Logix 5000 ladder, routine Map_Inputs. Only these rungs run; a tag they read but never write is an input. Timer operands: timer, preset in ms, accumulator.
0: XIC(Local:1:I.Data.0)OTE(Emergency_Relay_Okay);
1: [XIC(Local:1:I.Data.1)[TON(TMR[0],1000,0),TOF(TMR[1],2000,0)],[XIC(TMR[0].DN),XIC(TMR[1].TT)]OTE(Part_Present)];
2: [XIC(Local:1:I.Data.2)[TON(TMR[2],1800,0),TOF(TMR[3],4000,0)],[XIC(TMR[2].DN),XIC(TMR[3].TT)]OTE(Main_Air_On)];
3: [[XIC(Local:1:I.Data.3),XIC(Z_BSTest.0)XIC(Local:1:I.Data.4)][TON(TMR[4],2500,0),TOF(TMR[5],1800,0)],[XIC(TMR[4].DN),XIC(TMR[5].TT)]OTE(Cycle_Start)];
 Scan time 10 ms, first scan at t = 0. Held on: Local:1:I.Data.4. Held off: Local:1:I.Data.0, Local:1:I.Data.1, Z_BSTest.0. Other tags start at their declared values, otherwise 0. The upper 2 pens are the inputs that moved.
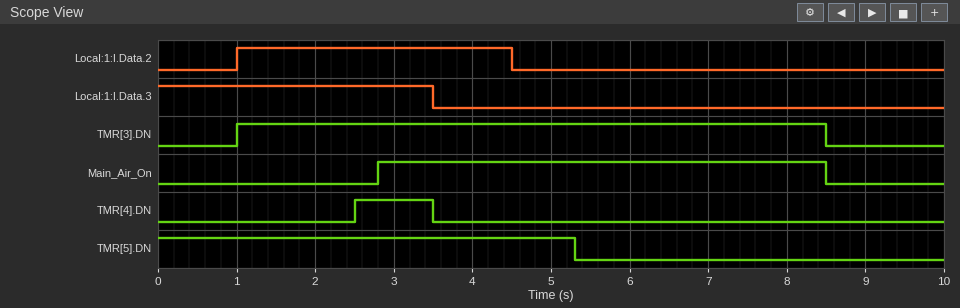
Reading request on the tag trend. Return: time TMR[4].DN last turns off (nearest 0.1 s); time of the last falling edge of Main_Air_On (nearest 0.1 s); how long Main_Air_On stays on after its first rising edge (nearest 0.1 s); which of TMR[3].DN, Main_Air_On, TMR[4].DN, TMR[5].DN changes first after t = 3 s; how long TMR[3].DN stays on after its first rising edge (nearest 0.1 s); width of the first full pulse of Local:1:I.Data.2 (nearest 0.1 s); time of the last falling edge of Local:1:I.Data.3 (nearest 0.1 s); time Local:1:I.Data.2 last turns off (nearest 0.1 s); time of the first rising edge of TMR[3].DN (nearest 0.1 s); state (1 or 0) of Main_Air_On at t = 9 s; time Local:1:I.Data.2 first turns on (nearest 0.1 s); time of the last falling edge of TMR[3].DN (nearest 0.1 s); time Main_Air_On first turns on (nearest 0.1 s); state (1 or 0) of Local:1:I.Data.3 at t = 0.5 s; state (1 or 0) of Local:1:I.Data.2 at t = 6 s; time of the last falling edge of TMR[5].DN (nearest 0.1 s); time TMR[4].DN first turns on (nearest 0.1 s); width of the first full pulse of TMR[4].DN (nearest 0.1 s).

3.5 s
8.5 s
5.7 s
TMR[4].DN
7.5 s
3.5 s
3.5 s
4.5 s
1.0 s
0
1.0 s
8.5 s
2.8 s
1
0
5.3 s
2.5 s
1.0 s
